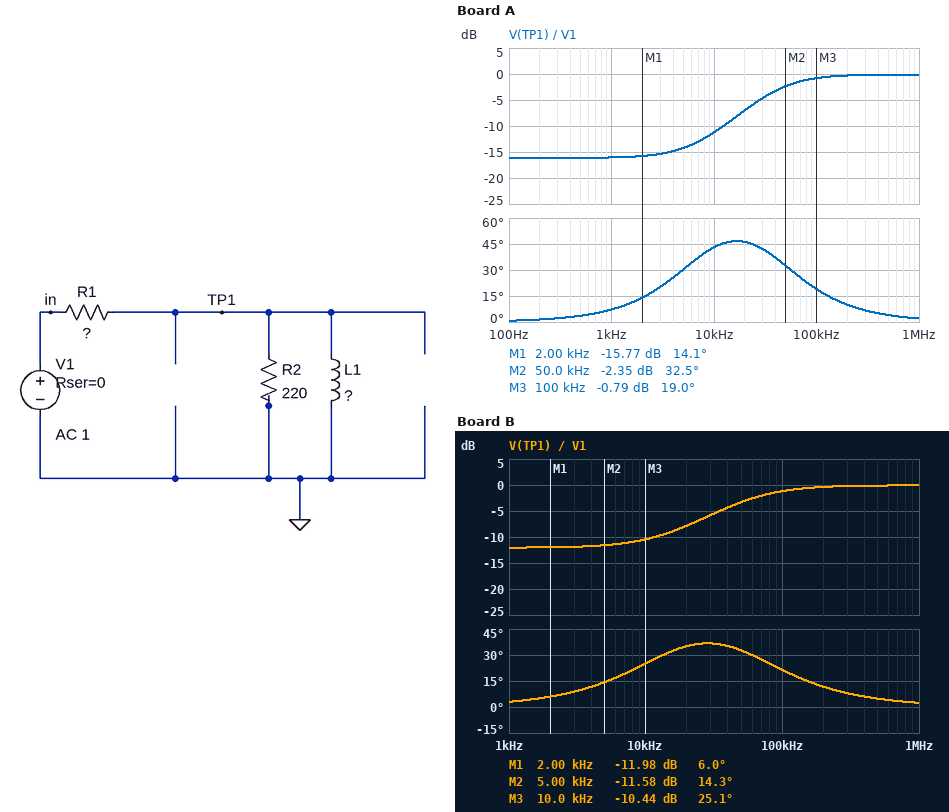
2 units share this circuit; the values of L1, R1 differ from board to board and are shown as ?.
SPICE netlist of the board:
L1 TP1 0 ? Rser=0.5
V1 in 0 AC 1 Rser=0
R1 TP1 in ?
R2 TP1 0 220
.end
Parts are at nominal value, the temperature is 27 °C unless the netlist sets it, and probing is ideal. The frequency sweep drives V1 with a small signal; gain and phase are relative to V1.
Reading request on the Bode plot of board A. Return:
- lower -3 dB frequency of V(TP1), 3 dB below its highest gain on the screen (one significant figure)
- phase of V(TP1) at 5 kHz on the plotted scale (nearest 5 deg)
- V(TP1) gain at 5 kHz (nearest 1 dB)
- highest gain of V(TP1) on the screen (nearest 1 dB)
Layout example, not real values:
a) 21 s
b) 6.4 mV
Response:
a) 40 kHz
b) 30 deg
c) -14 dB
d) 0 dB
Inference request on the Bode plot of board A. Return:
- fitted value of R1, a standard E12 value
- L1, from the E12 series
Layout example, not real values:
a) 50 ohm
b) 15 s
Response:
a) 2.7 Ω
b) 12 µH
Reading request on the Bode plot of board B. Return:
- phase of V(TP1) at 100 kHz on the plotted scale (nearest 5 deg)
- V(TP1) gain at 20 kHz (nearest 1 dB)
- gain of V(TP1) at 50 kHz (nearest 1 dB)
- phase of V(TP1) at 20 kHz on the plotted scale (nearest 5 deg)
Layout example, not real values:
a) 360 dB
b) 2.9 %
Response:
a) 20 deg
b) -8 dB
c) -3 dB
d) 35 deg
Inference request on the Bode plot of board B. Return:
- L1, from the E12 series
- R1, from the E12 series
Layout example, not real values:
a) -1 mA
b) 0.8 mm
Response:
a) 5.6 µH
b) 1.5 Ω
